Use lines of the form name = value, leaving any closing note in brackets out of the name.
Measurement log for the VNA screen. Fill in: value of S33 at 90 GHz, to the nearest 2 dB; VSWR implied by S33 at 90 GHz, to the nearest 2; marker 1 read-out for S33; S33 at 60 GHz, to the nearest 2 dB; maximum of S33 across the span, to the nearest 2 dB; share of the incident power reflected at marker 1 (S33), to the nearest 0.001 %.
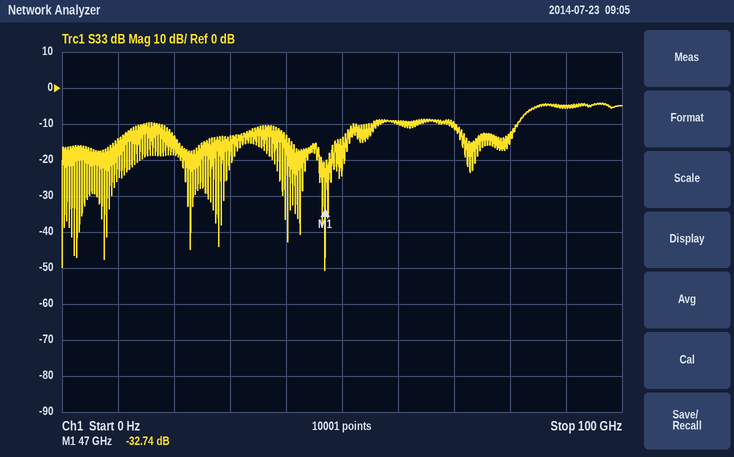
value of S33 at 90 GHz, to the nearest 2 dB = -4 dB
VSWR implied by S33 at 90 GHz, to the nearest 2 = 4
marker 1 read-out for S33 = -32.74 dB
S33 at 60 GHz, to the nearest 2 dB = -10 dB
maximum of S33 across the span, to the nearest 2 dB = -4 dB
share of the incident power reflected at marker 1 (S33), to the nearest 0.001 % = 0.053 %
